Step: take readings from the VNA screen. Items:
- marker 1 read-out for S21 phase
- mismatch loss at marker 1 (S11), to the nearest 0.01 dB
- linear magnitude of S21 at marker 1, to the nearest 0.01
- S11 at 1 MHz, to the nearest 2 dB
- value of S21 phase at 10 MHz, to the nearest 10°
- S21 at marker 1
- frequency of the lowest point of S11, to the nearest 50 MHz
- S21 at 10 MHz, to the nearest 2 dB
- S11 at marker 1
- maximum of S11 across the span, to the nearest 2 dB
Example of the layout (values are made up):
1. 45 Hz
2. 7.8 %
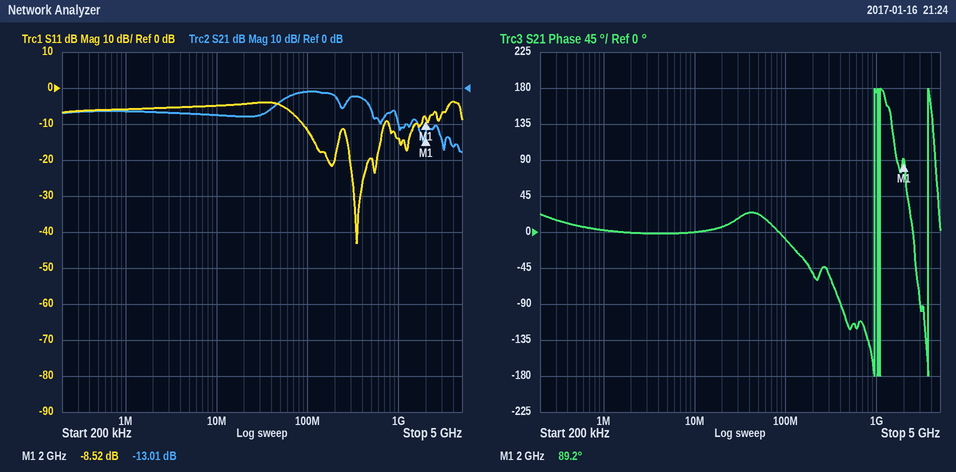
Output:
1. 89.2°
2. 0.66 dB
3. 0.22
4. -6 dB
5. 0°
6. -13.01 dB
7. 350 MHz
8. -8 dB
9. -8.52 dB
10. -4 dB
